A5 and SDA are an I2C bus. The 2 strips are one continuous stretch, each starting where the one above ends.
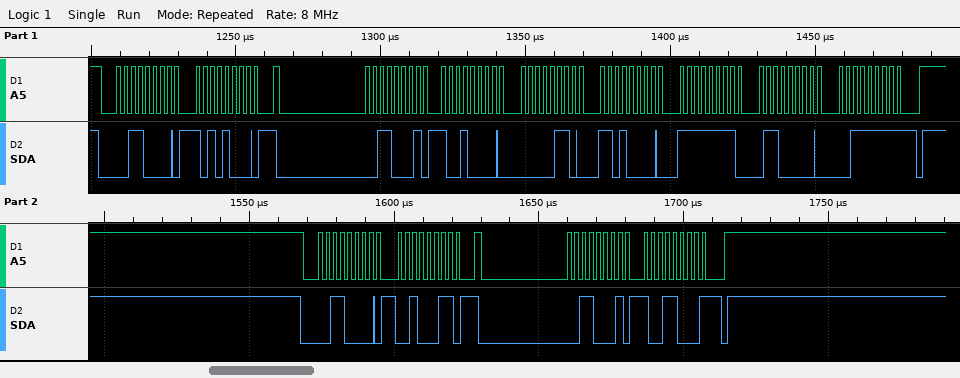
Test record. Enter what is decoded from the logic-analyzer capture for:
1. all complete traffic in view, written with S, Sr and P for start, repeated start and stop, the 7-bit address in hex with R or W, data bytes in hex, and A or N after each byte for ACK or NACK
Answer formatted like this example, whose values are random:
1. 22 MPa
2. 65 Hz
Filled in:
1. S 18W A A8 A Sr 18R A 90 A 06 A D0 A FF A 60 A 3F N P S 18W A 23 A Sr 18R A 98 N P
